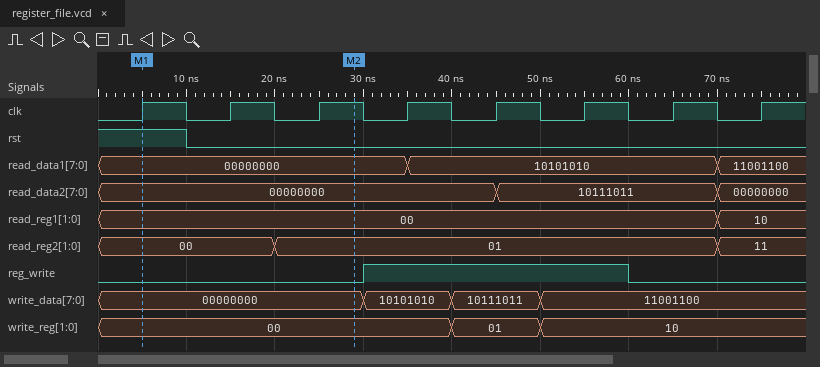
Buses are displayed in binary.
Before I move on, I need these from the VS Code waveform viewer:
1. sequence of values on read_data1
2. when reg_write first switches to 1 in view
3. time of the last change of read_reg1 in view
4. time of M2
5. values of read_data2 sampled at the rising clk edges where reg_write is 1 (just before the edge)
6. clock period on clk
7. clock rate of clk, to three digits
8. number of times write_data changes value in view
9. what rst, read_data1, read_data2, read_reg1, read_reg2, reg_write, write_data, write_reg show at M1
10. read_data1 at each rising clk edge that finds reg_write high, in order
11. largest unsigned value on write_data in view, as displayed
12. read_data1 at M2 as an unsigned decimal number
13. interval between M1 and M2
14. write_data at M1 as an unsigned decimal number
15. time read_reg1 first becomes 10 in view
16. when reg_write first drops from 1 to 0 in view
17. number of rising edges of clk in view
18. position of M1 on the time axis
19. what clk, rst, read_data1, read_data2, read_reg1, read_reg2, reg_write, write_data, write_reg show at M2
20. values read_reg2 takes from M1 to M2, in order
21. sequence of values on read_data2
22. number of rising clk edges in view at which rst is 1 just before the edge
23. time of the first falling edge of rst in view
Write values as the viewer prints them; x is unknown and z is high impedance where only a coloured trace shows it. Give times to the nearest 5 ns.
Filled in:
00000000, 10101010, 11001100
30 ns
70 ns
30 ns
00000000, 00000000, 10111011
10 ns
100 MHz
3
rst=1, read_data1=00000000, read_data2=00000000, read_reg1=00, read_reg2=00, reg_write=0, write_data=00000000, write_reg=00
00000000, 10101010, 10101010
11001100
0
25 ns
0
70 ns
60 ns
8
5 ns
clk=1, rst=0, read_data1=00000000, read_data2=00000000, read_reg1=00, read_reg2=01, reg_write=0, write_data=00000000, write_reg=00
00, 01
00000000, 10111011, 00000000
1
10 ns
